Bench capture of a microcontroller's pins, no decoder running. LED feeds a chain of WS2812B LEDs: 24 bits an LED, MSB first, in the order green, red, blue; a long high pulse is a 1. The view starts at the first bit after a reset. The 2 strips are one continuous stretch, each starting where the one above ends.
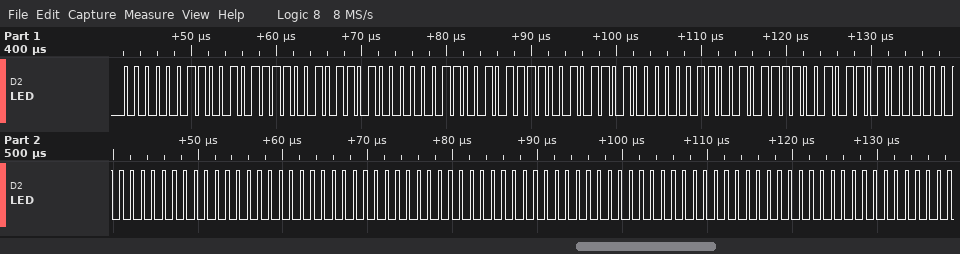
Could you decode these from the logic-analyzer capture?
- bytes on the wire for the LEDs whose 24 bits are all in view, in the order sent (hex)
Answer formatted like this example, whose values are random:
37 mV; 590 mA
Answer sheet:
03 2F 2D 03 2F 2D 03 2F 2D 00 00 00 00 00 00 00 00 00
